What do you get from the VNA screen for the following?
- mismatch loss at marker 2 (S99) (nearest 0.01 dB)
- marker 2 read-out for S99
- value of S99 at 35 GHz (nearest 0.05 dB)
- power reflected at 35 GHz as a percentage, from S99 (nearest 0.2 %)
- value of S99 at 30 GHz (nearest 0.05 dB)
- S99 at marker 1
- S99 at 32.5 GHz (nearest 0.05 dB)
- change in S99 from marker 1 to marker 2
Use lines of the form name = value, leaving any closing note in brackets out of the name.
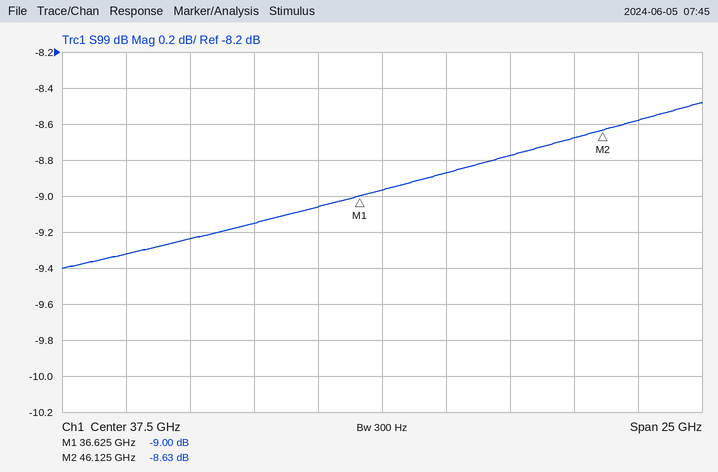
mismatch loss at marker 2 (S99) = 0.64 dB
marker 2 read-out for S99 = -8.63 dB
value of S99 at 35 GHz = -9.05 dB
power reflected at 35 GHz as a percentage, from S99 = 12.4 %
value of S99 at 30 GHz = -9.25 dB
S99 at marker 1 = -9.00 dB
S99 at 32.5 GHz = -9.15 dB
change in S99 from marker 1 to marker 2 = 0.37 dB
